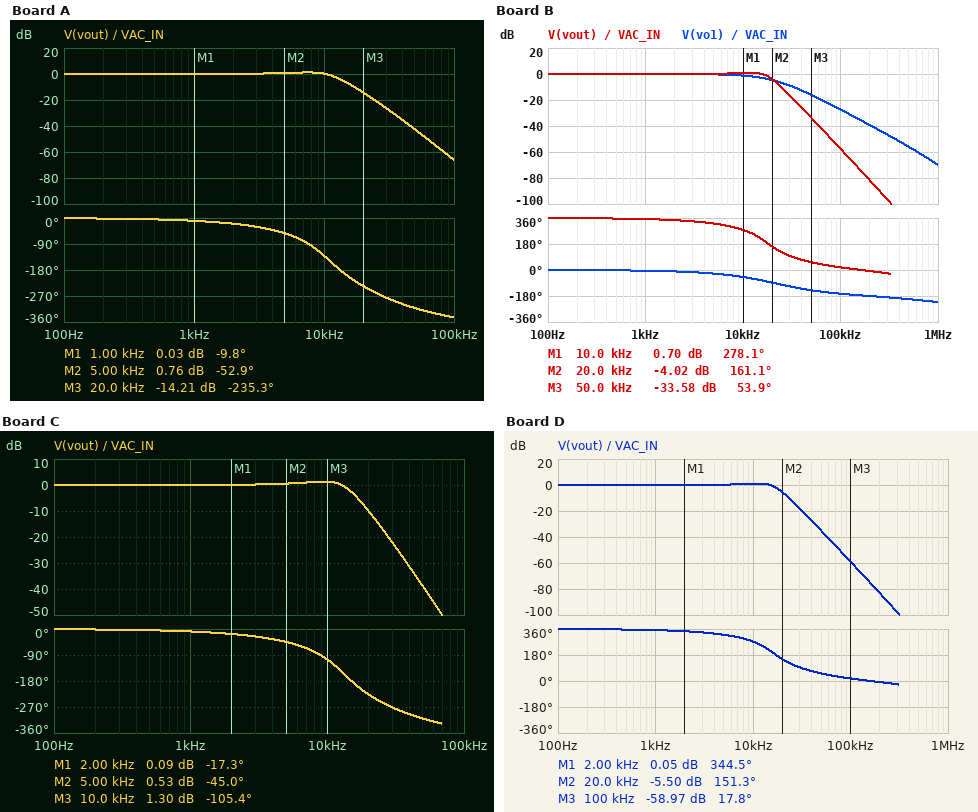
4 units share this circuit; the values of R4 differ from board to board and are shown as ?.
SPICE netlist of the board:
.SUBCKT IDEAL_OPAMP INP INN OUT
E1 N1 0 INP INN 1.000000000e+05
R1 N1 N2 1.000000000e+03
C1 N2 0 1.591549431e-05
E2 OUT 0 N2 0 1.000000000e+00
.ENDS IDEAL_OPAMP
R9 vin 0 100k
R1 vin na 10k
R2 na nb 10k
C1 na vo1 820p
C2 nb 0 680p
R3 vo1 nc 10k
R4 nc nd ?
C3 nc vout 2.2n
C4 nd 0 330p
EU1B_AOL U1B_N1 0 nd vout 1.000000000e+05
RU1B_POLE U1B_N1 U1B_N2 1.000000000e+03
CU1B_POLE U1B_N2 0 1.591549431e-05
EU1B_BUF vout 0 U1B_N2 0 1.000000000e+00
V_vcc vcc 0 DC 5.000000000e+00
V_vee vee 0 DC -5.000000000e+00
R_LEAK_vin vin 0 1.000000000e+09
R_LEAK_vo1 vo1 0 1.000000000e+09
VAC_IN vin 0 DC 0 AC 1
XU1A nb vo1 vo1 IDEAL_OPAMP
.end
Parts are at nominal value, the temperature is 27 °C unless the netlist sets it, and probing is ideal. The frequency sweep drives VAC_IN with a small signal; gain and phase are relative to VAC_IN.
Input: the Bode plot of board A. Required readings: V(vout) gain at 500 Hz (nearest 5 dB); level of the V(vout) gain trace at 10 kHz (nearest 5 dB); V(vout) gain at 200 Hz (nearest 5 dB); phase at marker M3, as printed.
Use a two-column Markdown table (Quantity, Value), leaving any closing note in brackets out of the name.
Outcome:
| Quantity | Value |
|---|---|
| V(vout) gain at 500 Hz | 0 dB |
| level of the V(vout) gain trace at 10 kHz | 0 dB |
| V(vout) gain at 200 Hz | 0 dB |
| phase at marker M3, as printed | -235.3 deg |
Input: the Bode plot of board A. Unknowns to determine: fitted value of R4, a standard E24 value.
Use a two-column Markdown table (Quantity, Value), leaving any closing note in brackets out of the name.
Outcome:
| Quantity | Value |
|---|---|
| fitted value of R4, a standard E24 value | 30 kΩ |
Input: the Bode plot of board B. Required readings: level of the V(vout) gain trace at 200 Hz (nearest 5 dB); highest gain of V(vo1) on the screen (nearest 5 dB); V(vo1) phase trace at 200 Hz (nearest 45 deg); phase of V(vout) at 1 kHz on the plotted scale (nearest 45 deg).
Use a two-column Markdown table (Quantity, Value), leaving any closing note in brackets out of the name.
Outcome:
| Quantity | Value |
|---|---|
| level of the V(vout) gain trace at 200 Hz | 0 dB |
| highest gain of V(vo1) on the screen | 0 dB |
| V(vo1) phase trace at 200 Hz | 0 deg |
| phase of V(vout) at 1 kHz on the plotted scale | 360 deg |
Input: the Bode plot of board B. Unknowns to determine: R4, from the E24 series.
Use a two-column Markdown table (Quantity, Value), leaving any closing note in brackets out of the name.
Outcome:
| Quantity | Value |
|---|---|
| R4, from the E24 series | 11 kΩ |
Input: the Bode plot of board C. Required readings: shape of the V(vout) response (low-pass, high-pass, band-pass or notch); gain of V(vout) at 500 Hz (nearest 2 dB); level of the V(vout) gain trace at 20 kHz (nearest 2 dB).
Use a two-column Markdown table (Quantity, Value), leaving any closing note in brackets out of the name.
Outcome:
| Quantity | Value |
|---|---|
| shape of the V(vout) response | low-pass |
| gain of V(vout) at 500 Hz | 0 dB |
| level of the V(vout) gain trace at 20 kHz | -10 dB |
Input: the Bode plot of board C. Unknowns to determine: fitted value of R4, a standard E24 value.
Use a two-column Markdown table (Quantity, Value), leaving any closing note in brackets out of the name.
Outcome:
| Quantity | Value |
|---|---|
| fitted value of R4, a standard E24 value | 20 kΩ |
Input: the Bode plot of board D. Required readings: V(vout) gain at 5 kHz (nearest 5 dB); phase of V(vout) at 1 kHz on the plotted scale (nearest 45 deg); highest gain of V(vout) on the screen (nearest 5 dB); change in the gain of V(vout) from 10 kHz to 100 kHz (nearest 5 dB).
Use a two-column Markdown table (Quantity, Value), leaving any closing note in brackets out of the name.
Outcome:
| Quantity | Value |
|---|---|
| V(vout) gain at 5 kHz | 0 dB |
| phase of V(vout) at 1 kHz on the plotted scale | 360 deg |
| highest gain of V(vout) on the screen | 0 dB |
| change in the gain of V(vout) from 10 kHz to 100 kHz | -60 dB |
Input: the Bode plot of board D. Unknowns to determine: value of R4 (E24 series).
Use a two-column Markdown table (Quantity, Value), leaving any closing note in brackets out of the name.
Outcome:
| Quantity | Value |
|---|---|
| value of R4 | 13 kΩ |
